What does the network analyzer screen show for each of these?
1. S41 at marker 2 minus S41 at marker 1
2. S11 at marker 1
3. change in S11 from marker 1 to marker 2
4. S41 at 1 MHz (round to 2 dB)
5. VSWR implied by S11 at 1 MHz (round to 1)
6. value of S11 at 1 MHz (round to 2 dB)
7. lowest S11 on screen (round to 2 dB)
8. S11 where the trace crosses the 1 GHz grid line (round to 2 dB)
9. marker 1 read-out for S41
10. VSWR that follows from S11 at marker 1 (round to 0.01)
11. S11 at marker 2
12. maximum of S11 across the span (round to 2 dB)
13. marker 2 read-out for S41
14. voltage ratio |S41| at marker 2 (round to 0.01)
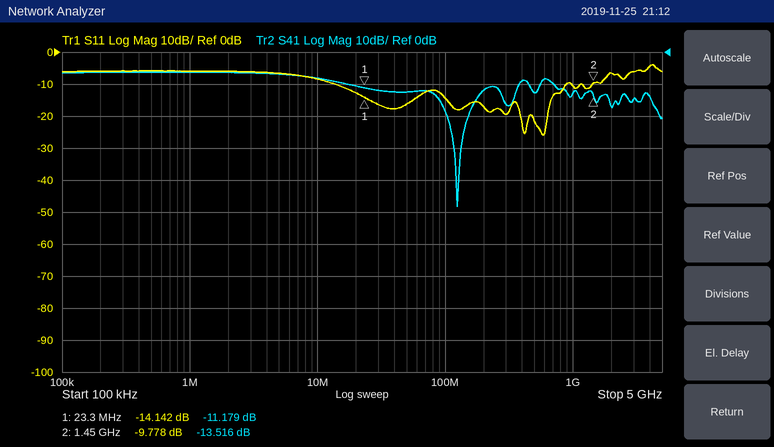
-2.337 dB
-14.142 dB
4.364 dB
-6 dB
3
-6 dB
-26 dB
-10 dB
-11.179 dB
1.49
-9.778 dB
-4 dB
-13.516 dB
0.21
